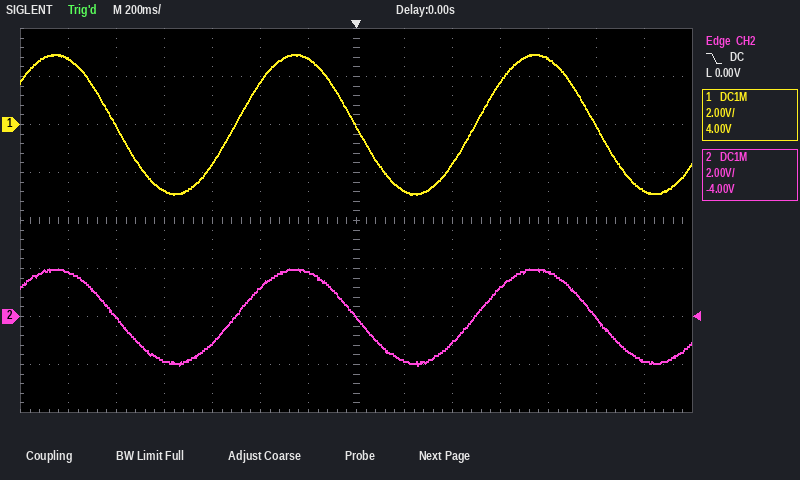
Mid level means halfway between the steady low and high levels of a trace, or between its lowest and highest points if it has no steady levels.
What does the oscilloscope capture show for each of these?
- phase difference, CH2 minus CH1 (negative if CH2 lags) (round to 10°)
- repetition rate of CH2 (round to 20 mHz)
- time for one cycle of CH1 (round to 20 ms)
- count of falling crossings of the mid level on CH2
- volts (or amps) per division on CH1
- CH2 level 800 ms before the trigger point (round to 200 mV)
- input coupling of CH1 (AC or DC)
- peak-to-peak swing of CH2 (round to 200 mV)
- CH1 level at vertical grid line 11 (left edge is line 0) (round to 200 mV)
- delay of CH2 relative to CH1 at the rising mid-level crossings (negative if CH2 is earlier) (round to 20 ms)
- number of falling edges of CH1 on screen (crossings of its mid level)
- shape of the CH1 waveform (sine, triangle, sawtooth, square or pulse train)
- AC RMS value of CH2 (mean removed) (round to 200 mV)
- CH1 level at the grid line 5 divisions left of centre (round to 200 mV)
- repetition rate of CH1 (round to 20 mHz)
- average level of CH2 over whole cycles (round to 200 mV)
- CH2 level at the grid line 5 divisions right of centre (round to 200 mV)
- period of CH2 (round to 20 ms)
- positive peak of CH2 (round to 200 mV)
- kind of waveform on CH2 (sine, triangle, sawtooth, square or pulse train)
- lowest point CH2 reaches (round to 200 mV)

0°
1.00 Hz
1.00 s
3
2 V
-1.8 V
DC
4.0 V
2.8 V
0 ms
3
sine
1.4 V
0.0 V
1.00 Hz
0.0 V
0.0 V
1.00 s
2.0 V
sine
-2.0 V
